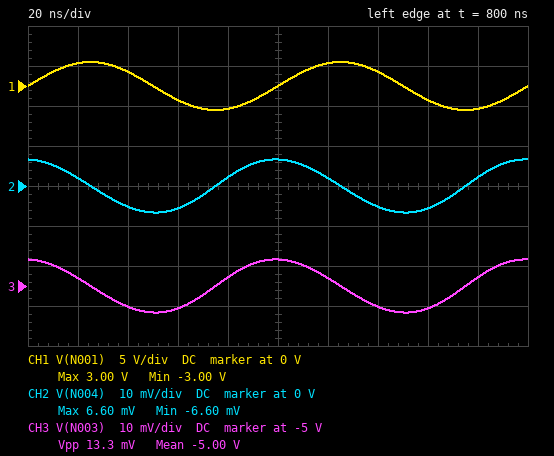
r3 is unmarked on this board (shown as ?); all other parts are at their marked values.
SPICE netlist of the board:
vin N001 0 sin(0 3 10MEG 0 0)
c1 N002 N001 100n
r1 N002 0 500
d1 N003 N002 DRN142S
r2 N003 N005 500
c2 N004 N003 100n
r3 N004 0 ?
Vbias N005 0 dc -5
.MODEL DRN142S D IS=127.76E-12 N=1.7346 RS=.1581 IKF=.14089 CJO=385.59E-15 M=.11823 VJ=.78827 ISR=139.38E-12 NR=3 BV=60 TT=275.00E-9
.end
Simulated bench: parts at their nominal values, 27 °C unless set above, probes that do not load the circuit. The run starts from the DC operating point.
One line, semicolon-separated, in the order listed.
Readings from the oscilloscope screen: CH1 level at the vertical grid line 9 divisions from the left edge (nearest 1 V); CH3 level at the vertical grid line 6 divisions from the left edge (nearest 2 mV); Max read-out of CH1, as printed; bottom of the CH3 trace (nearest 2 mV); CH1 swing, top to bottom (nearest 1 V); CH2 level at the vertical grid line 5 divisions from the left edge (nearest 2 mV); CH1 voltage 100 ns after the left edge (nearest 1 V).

-3 V; -4.998 V; 3.00 V; -5.006 V; 6 V; 6 mV; 0 V
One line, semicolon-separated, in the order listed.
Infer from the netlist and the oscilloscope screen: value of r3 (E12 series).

150 Ω
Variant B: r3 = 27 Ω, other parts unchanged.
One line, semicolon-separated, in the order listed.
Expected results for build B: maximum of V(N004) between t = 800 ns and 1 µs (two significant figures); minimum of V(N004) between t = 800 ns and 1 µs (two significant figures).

1.5 mV; -1.5 mV
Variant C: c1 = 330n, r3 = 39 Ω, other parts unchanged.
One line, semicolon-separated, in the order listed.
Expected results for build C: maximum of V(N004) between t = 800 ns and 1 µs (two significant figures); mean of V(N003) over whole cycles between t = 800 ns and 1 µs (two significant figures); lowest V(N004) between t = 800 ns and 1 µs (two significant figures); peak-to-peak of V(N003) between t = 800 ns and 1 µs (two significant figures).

2.1 mV; -5.0 V; -2.1 mV; 4.2 mV
